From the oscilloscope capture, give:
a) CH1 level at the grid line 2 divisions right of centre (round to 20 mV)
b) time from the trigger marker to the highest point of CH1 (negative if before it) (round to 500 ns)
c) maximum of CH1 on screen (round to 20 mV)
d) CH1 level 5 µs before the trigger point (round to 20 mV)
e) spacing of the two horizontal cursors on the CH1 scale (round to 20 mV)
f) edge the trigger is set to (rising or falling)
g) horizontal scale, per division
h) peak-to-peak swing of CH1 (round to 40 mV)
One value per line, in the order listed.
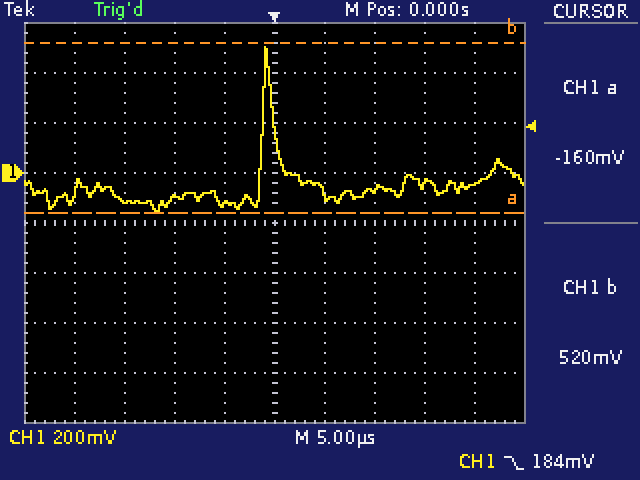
-60 mV
-1.0 µs
500 mV
-120 mV
680 mV
falling
5 µs
640 mV
